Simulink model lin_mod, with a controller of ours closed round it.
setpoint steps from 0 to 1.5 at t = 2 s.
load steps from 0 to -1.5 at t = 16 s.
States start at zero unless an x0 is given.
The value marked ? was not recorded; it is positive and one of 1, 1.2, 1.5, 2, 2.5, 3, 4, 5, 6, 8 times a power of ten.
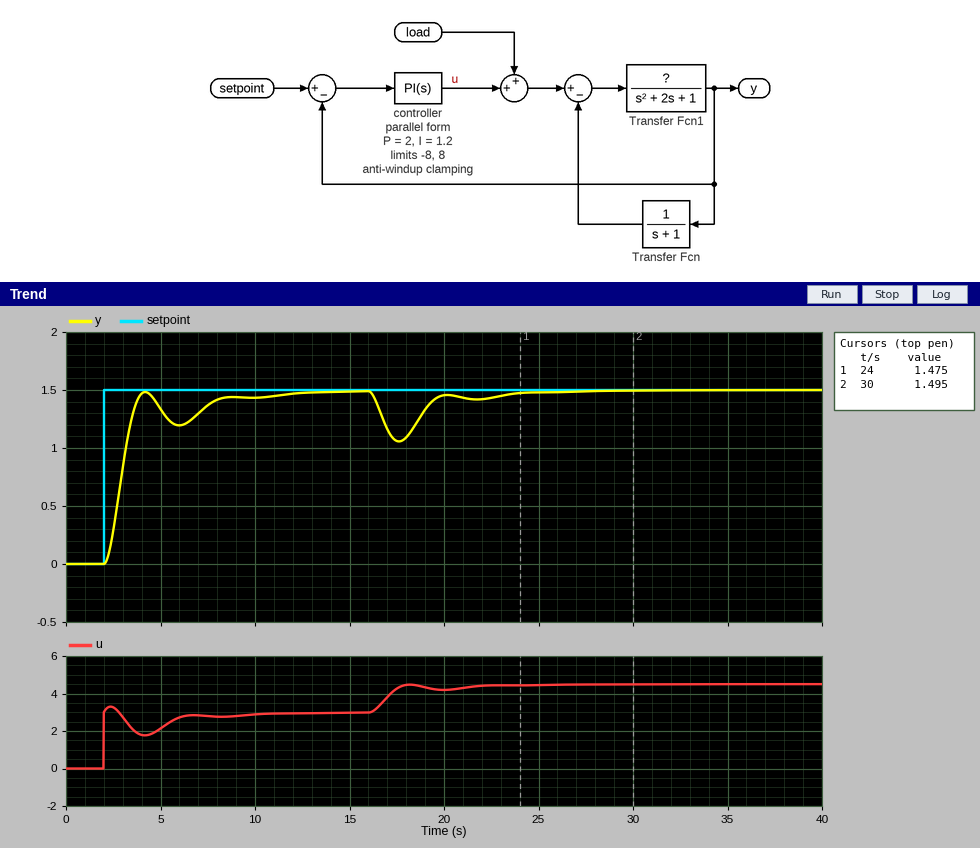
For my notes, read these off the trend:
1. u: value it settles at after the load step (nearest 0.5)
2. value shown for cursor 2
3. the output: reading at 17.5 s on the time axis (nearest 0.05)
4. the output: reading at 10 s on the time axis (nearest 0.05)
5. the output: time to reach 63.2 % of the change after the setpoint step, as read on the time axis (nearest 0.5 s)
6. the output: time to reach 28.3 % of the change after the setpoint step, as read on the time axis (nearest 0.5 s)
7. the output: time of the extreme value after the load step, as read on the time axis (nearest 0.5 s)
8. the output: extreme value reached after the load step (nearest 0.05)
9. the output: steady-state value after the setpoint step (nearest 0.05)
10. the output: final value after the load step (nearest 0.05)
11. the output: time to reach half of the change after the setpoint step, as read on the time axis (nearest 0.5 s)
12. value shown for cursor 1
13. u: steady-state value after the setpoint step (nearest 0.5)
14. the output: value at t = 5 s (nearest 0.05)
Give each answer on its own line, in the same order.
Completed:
4.5
1.495
1.05
1.45
3.0 s
2.5 s
17.5 s
1.05
1.50
1.50
3.0 s
1.475
3.0
1.35
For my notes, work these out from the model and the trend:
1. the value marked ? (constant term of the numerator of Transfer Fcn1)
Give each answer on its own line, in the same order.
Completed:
1
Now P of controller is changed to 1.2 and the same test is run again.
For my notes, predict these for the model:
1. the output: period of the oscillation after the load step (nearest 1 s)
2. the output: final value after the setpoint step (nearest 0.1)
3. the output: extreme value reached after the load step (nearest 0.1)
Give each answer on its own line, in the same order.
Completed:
5 s
1.5
1.0
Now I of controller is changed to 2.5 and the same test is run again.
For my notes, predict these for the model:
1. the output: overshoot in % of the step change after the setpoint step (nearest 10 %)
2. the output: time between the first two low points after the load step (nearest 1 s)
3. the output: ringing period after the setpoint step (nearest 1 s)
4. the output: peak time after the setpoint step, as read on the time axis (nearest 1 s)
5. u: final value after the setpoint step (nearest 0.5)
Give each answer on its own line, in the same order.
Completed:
30 %
4 s
4 s
4 s
3.0
